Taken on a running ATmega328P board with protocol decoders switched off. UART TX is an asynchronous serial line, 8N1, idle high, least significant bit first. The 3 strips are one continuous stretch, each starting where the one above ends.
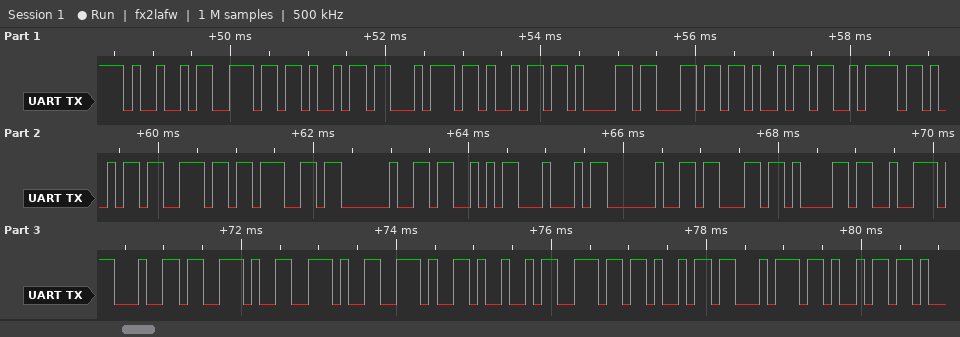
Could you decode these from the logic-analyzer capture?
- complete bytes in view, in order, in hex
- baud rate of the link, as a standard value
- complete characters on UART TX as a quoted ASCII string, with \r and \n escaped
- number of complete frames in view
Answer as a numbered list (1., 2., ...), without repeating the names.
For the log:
1. 0x49 0x6E 0x69 0x74 0x69 0x61 0x6C 0x69 0x7A 0x69 0x6E 0x67 0x20 0x53 0x44 0x20 0x63 0x61 0x72 0x64 0x2E 0x2E 0x2E 0x49 0x6E 0x69 0x74 0x69
2. 9600 baud
3. "Initializing SD card...Initi"
4. 28
